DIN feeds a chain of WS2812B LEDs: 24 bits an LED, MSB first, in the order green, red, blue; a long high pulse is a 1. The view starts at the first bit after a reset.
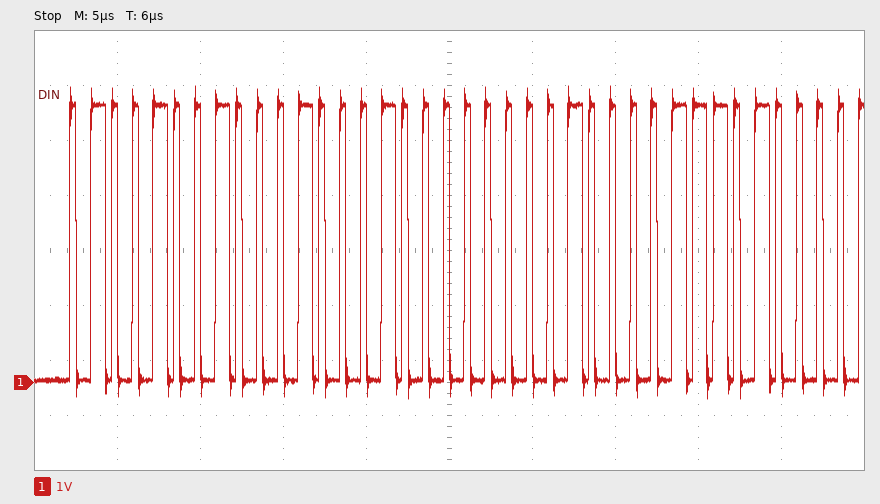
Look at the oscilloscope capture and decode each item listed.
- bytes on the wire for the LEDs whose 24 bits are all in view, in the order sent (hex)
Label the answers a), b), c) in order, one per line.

a) 49 11 00
